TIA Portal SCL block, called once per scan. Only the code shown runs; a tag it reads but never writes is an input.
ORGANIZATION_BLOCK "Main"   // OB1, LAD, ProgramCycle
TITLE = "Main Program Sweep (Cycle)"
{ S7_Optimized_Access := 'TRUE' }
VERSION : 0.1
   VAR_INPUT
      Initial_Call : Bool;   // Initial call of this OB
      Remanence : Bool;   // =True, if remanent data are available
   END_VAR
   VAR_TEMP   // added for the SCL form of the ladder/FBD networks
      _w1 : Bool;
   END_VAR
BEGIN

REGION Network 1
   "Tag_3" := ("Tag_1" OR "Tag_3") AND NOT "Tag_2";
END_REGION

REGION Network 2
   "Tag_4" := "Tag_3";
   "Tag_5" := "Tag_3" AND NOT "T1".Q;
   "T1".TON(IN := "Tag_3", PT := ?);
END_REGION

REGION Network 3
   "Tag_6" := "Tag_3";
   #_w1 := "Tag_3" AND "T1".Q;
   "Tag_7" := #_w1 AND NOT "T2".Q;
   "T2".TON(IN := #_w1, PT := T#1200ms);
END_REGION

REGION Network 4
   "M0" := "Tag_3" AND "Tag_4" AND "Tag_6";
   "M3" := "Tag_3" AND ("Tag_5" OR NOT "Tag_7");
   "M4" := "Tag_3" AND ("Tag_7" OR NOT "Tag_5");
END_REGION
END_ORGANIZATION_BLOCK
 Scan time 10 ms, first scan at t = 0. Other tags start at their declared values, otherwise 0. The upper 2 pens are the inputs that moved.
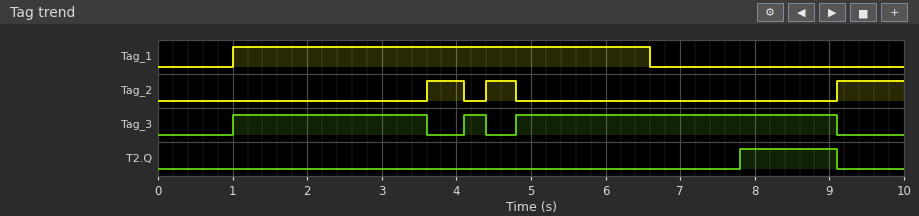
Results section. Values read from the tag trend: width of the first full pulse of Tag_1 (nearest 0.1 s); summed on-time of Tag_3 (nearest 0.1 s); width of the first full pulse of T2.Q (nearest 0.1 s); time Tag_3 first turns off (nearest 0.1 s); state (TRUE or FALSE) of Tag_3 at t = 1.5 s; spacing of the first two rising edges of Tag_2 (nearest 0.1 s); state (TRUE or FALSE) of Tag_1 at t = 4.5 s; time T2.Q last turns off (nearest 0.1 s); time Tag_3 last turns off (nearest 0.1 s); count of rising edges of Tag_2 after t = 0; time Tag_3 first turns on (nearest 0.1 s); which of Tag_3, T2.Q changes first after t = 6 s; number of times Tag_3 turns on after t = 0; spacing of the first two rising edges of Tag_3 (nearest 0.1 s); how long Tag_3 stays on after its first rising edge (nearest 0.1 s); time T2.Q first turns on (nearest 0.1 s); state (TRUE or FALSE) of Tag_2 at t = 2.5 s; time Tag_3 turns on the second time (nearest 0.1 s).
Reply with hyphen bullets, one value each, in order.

- 5.6 s
- 7.2 s
- 1.3 s
- 3.6 s
- TRUE
- 0.8 s
- TRUE
- 9.1 s
- 9.1 s
- 3
- 1.0 s
- T2.Q
- 3
- 3.1 s
- 2.6 s
- 7.8 s
- FALSE
- 4.1 s
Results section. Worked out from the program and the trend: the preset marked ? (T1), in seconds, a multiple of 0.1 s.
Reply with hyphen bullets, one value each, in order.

- 1.8 s
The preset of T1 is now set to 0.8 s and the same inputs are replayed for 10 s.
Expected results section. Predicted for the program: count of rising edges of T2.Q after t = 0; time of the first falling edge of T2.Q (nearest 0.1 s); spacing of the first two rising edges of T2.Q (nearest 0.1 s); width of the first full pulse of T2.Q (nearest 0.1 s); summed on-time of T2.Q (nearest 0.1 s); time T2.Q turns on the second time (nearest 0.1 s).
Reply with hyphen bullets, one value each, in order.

- 2
- 3.6 s
- 3.8 s
- 0.6 s
- 2.9 s
- 6.8 s
